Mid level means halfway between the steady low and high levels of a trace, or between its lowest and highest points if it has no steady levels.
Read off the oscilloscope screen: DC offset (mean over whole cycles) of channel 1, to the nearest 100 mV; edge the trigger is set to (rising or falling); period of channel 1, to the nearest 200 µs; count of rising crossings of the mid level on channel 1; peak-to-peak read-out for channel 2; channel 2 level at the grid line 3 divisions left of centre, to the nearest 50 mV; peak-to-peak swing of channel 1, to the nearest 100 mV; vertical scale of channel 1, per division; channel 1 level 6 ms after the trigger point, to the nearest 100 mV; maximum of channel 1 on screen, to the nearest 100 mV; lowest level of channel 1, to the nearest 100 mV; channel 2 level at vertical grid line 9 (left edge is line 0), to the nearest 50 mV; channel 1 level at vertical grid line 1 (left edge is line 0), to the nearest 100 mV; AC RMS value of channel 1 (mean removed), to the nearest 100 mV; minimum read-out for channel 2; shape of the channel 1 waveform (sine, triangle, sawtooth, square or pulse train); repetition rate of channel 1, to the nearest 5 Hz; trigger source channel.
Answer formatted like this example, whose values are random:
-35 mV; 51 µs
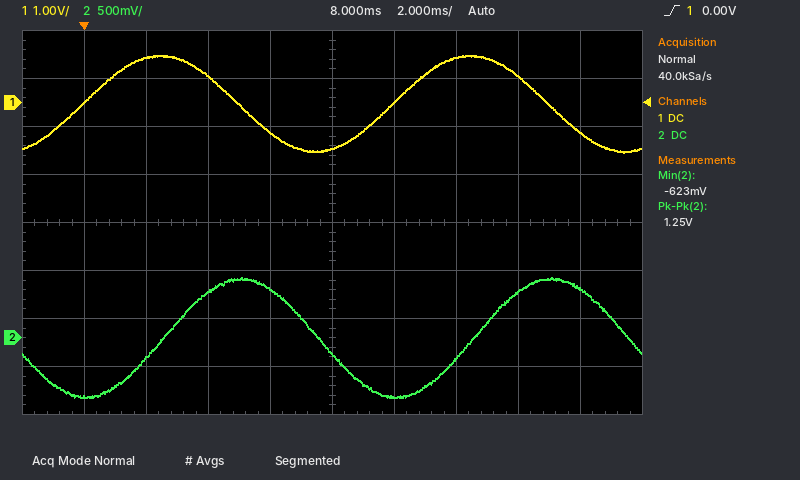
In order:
0.0 V; rising; 10.0 ms; 2; 1.25 V; -200 mV; 2.0 V; 1 V; -600 mV; 1.0 V; -1.0 V; 500 mV; 0.0 V; 700 mV; -623 mV; sine; 100 Hz; channel 1
